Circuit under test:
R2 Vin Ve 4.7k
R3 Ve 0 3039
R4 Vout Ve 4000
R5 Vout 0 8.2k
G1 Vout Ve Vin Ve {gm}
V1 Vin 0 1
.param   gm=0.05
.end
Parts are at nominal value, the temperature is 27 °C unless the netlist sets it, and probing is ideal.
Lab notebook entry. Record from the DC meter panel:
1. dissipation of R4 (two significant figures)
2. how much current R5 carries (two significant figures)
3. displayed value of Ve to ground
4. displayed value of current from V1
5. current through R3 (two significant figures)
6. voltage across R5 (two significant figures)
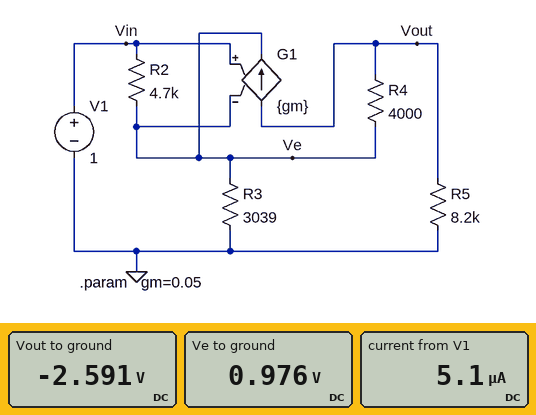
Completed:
3.2 mW
320 µA
0.976 V
5.1 µA
320 µA
2.6 V
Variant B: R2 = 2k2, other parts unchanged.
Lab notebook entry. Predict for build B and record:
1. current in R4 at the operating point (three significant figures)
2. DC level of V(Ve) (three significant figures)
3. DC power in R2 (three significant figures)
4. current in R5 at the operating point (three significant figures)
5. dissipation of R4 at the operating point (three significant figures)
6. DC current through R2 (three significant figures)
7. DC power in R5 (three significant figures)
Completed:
880 µA
976 mV
258 nW
310 µA
3.10 mW
10.8 µA
790 µW
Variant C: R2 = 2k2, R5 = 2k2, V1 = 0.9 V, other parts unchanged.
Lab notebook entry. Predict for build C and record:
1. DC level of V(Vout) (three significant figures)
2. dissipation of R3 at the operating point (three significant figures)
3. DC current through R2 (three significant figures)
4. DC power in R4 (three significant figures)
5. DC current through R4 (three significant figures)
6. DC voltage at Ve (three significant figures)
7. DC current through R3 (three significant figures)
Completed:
-629 mV
259 µW
6.04 µA
574 µW
379 µA
887 mV
292 µA
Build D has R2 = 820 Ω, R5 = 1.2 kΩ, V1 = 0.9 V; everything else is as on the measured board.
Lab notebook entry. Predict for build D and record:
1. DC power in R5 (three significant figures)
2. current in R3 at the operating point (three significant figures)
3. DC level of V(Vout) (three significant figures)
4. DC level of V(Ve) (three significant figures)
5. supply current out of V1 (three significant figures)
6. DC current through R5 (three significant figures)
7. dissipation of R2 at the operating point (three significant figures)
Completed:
92.8 µW
292 µA
-334 mV
888 mV
14.2 µA
278 µA
166 nW
